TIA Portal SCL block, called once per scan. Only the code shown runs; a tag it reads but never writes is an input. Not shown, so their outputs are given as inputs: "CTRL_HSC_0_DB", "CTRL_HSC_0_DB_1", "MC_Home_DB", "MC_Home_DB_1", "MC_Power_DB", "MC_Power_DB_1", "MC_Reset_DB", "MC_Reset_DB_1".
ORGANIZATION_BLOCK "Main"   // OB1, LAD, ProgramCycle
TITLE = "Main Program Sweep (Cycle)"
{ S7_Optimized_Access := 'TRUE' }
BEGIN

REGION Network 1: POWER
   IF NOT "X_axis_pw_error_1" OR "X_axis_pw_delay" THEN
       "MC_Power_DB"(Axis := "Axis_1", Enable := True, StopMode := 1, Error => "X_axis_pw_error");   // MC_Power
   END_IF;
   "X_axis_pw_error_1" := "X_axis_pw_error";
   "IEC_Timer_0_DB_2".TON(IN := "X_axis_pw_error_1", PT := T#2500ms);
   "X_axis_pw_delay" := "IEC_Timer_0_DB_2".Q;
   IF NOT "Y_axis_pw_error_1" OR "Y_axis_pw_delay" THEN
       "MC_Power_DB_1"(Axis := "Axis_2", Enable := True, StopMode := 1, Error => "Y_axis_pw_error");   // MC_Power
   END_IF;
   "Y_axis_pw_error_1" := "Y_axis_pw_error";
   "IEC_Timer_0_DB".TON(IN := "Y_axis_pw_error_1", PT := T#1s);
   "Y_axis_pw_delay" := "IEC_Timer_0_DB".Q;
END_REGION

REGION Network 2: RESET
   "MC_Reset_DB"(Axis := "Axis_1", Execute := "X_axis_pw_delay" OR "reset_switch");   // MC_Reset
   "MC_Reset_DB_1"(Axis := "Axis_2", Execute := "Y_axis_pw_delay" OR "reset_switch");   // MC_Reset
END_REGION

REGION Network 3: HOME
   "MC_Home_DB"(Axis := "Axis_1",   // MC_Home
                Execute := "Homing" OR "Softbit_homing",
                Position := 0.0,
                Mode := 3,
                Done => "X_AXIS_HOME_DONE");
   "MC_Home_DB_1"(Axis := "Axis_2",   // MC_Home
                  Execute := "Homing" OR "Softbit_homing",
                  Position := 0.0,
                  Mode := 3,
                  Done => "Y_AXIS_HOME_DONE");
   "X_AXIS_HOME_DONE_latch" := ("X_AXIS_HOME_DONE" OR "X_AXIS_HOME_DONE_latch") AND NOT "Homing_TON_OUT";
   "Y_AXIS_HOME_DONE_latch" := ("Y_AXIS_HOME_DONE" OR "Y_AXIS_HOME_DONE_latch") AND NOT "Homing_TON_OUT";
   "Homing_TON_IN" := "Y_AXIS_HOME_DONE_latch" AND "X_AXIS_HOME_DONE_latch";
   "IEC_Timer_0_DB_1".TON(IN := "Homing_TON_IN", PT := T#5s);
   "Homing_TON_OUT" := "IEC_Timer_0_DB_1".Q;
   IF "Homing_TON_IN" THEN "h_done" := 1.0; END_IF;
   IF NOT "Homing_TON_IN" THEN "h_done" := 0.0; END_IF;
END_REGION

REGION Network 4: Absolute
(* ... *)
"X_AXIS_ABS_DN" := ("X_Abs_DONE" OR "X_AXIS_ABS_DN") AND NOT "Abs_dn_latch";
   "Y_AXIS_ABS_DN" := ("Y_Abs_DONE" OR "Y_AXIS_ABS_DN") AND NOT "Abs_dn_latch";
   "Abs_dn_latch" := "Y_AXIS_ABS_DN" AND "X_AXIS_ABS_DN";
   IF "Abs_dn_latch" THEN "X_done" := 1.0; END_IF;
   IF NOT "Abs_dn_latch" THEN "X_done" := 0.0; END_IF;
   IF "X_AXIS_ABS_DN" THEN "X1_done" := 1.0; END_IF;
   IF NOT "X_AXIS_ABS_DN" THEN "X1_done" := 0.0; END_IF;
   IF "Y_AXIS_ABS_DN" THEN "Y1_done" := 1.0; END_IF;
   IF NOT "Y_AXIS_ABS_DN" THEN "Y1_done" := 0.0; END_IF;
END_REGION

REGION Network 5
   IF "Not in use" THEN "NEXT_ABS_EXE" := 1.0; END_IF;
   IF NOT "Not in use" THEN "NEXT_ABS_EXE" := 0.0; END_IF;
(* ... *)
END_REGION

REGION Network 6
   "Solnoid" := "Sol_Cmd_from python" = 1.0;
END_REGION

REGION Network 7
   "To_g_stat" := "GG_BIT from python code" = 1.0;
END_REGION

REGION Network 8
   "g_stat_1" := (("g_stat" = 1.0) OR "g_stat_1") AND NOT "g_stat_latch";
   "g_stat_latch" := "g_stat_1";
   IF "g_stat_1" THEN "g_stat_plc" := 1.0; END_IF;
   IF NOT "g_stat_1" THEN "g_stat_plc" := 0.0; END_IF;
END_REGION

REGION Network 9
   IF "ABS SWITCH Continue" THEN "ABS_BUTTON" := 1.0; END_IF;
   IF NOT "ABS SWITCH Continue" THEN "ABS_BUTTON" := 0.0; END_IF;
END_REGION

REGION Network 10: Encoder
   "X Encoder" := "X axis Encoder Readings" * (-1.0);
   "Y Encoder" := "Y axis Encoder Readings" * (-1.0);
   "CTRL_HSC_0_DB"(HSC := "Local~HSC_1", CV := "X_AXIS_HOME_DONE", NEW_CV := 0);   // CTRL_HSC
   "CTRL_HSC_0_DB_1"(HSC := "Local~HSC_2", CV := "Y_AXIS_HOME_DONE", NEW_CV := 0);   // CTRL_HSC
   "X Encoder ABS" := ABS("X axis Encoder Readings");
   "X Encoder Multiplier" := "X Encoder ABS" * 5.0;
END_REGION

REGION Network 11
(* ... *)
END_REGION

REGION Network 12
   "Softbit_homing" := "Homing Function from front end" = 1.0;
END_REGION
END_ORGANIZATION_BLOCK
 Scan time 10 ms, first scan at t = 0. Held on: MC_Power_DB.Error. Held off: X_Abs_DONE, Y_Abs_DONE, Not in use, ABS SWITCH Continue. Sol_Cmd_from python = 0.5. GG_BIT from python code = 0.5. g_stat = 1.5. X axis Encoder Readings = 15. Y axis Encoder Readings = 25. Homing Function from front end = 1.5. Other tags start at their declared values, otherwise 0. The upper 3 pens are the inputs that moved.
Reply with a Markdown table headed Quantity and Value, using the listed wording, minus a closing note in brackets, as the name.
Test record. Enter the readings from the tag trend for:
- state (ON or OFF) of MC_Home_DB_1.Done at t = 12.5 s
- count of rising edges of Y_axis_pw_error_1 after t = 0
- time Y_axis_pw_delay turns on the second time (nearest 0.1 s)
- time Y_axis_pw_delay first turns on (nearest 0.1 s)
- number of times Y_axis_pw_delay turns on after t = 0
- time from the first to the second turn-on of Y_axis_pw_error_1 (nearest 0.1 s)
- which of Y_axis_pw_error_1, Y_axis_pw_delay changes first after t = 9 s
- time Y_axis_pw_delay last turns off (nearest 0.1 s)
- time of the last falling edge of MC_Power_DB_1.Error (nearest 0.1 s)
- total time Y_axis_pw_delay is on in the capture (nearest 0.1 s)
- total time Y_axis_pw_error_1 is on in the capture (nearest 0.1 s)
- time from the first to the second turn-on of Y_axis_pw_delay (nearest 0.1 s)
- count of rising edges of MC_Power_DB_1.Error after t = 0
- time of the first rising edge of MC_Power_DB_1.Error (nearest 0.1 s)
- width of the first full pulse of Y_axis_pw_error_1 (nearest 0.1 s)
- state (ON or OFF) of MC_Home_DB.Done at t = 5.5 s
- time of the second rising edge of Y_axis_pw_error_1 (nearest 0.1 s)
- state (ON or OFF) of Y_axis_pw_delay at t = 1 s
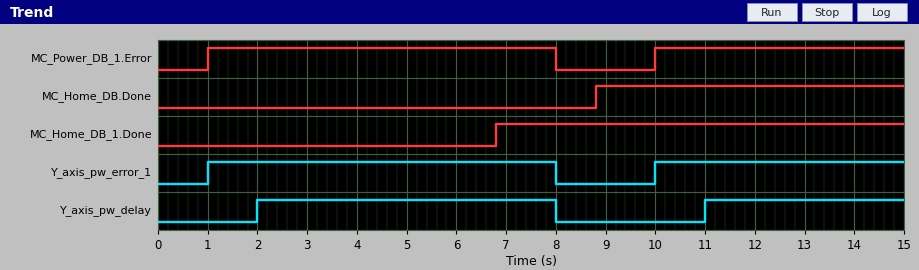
| Quantity | Value |
|---|---|
| state (ON or OFF) of MC_Home_DB_1.Done at t = 12.5 s | ON |
| count of rising edges of Y_axis_pw_error_1 after t = 0 | 2 |
| time Y_axis_pw_delay turns on the second time | 11.0 s |
| time Y_axis_pw_delay first turns on | 2.0 s |
| number of times Y_axis_pw_delay turns on after t = 0 | 2 |
| time from the first to the second turn-on of Y_axis_pw_error_1 | 9.0 s |
| which of Y_axis_pw_error_1, Y_axis_pw_delay changes first after t = 9 s | Y_axis_pw_error_1 |
| time Y_axis_pw_delay last turns off | 8.0 s |
| time of the last falling edge of MC_Power_DB_1.Error | 8.0 s |
| total time Y_axis_pw_delay is on in the capture | 10.0 s |
| total time Y_axis_pw_error_1 is on in the capture | 12.0 s |
| time from the first to the second turn-on of Y_axis_pw_delay | 9.0 s |
| count of rising edges of MC_Power_DB_1.Error after t = 0 | 2 |
| time of the first rising edge of MC_Power_DB_1.Error | 1.0 s |
| width of the first full pulse of Y_axis_pw_error_1 | 7.0 s |
| state (ON or OFF) of MC_Home_DB.Done at t = 5.5 s | OFF |
| time of the second rising edge of Y_axis_pw_error_1 | 10.0 s |
| state (ON or OFF) of Y_axis_pw_delay at t = 1 s | OFF |
